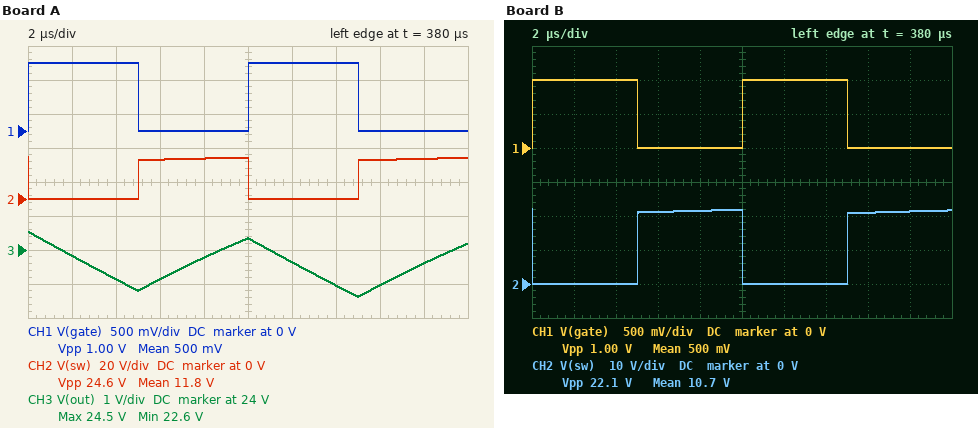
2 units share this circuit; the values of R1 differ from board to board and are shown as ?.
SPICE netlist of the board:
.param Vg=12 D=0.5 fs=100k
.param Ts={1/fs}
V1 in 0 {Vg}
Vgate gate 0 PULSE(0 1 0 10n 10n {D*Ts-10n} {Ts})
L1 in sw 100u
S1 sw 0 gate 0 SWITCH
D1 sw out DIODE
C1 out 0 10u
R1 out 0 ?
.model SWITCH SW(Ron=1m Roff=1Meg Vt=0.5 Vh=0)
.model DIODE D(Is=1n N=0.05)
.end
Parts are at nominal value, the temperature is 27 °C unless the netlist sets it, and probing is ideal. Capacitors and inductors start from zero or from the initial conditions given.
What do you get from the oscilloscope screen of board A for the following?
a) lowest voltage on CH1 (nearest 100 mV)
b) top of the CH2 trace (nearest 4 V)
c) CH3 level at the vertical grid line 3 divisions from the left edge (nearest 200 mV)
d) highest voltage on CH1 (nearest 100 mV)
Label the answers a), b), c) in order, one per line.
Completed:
a) 0 V
b) 24 V
c) 23.2 V
d) 1.0 V
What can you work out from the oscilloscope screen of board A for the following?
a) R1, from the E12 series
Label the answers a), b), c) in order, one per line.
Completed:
a) 6.8 Ω
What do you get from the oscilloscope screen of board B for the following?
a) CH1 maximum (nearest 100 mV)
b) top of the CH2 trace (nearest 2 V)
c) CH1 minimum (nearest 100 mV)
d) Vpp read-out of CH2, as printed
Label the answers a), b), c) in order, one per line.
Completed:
a) 1.0 V
b) 22 V
c) 0 V
d) 22.1 V
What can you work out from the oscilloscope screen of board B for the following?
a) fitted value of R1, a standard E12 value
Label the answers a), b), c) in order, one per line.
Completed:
a) 10 Ω
